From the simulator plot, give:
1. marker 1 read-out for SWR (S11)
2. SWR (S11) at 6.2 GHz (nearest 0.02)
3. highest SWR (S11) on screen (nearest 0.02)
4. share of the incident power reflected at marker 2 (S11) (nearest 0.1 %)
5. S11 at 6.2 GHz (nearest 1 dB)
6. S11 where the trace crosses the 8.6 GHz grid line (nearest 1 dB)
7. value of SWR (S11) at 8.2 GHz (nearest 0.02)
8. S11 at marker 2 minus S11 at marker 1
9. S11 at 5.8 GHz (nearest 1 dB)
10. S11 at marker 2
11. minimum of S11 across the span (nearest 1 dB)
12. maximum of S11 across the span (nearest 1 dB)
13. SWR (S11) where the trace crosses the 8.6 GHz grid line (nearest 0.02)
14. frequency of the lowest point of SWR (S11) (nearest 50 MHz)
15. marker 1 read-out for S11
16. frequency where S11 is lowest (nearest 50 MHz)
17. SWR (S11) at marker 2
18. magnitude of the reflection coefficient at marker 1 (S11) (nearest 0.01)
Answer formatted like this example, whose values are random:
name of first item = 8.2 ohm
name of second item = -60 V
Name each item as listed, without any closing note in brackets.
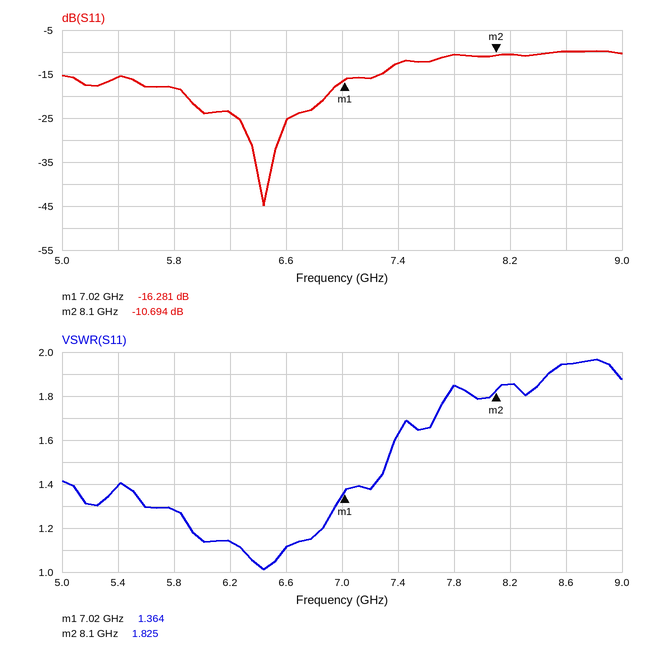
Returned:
marker 1 read-out for SWR = 1.364
SWR (S11) at 6.2 GHz = 1.14
highest SWR (S11) on screen = 1.96
share of the incident power reflected at marker 2 (S11) = 8.5 %
S11 at 6.2 GHz = -24 dB
S11 where the trace crosses the 8.6 GHz grid line = -10 dB
value of SWR (S11) at 8.2 GHz = 1.86
S11 at marker 2 minus S11 at marker 1 = 5.587 dB
S11 at 5.8 GHz = -18 dB
S11 at marker 2 = -10.694 dB
minimum of S11 across the span = -45 dB
maximum of S11 across the span = -10 dB
SWR (S11) where the trace crosses the 8.6 GHz grid line = 1.94
frequency of the lowest point of SWR (S11) = 6.45 GHz
marker 1 read-out for S11 = -16.281 dB
frequency where S11 is lowest = 6.45 GHz
SWR (S11) at marker 2 = 1.825
magnitude of the reflection coefficient at marker 1 (S11) = 0.15
